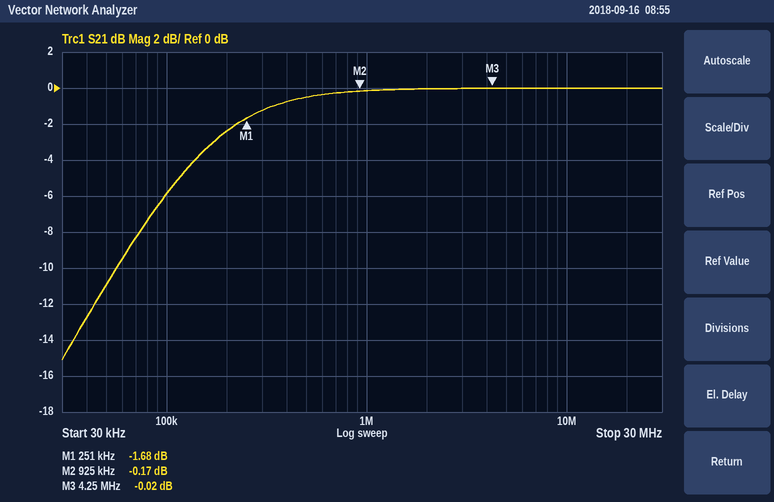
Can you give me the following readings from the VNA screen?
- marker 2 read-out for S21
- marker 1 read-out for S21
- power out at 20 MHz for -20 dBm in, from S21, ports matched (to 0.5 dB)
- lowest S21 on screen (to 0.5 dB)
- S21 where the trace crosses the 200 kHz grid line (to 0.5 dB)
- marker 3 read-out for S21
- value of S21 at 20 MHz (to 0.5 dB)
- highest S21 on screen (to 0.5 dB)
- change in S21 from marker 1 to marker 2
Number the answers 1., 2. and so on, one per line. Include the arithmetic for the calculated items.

1. -0.17 dB
2. -1.68 dB
3. -20 dBm + (0.0 dB) = -20.0 dBm
4. -15.0 dB
5. -2.5 dB
6. -0.02 dB
7. 0.0 dB
8. 0.0 dB
9. -0.17 − (-1.68) = 1.51 dB
